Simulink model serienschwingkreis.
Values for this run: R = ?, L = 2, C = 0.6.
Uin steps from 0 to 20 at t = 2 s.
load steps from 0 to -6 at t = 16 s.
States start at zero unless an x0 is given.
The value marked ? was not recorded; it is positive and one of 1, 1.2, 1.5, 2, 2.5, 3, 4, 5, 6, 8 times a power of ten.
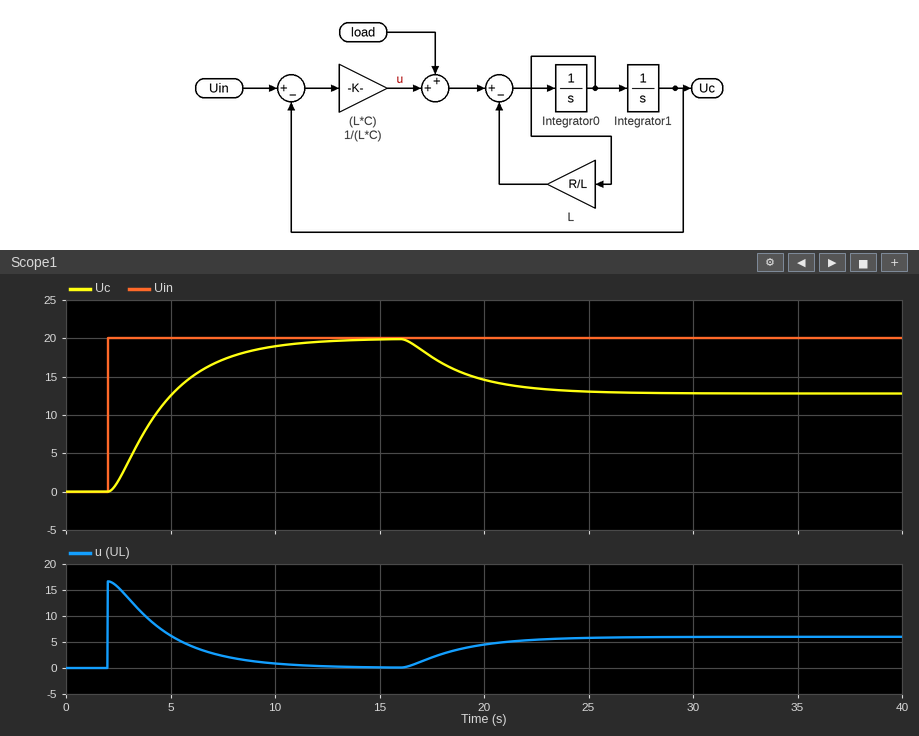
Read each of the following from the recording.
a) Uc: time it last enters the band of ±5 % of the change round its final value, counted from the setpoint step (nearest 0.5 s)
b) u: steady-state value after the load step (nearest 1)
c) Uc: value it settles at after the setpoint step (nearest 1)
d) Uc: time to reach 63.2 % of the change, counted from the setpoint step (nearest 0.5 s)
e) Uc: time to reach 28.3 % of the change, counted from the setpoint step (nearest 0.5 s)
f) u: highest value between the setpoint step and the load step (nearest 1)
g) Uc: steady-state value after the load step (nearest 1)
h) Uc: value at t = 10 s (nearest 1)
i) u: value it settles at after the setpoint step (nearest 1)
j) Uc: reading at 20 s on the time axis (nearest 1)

8.0 s
6
20
3.0 s
1.5 s
17
13
19
0
15
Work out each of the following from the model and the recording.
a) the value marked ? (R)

5
